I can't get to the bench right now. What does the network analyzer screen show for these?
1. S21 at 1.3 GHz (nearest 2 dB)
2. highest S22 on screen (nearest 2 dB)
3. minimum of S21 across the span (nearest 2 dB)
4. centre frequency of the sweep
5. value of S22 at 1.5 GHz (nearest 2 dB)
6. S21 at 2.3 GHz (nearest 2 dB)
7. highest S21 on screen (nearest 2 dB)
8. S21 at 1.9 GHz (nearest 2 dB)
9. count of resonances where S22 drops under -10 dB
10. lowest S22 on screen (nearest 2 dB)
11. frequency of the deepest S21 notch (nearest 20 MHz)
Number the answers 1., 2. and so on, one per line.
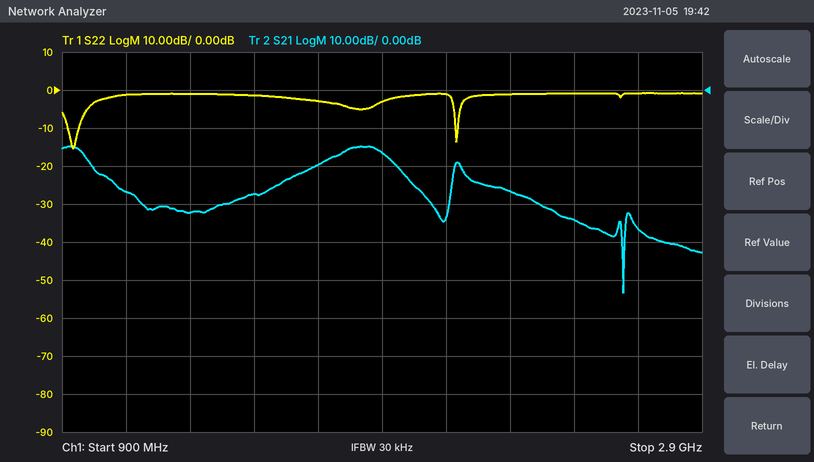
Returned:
1. -32 dB
2. 0 dB
3. -54 dB
4. 1.9 GHz
5. -2 dB
6. -26 dB
7. -14 dB
8. -16 dB
9. 2
10. -16 dB
11. 2.66 GHz
